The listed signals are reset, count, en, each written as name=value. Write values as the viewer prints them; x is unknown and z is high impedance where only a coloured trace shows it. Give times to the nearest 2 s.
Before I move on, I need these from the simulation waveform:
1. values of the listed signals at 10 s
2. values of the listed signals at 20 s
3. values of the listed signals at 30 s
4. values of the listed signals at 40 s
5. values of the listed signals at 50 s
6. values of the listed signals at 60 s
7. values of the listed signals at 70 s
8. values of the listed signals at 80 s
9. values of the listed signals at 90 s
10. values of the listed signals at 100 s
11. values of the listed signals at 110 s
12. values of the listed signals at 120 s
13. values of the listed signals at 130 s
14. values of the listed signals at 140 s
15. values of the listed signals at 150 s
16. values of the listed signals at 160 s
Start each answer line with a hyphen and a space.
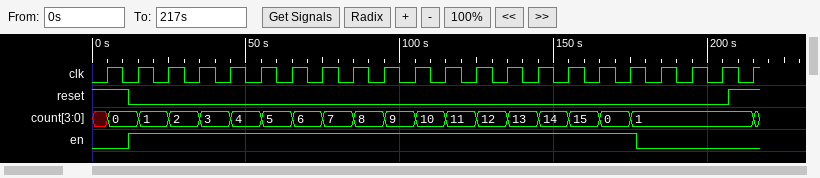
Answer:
- reset=1, count=0, en=0
- reset=0, count=1, en=1
- reset=0, count=2, en=1
- reset=0, count=3, en=1
- reset=0, count=4, en=1
- reset=0, count=5, en=1
- reset=0, count=6, en=1
- reset=0, count=7, en=1
- reset=0, count=8, en=1
- reset=0, count=9, en=1
- reset=0, count=10, en=1
- reset=0, count=11, en=1
- reset=0, count=12, en=1
- reset=0, count=13, en=1
- reset=0, count=14, en=1
- reset=0, count=15, en=1
